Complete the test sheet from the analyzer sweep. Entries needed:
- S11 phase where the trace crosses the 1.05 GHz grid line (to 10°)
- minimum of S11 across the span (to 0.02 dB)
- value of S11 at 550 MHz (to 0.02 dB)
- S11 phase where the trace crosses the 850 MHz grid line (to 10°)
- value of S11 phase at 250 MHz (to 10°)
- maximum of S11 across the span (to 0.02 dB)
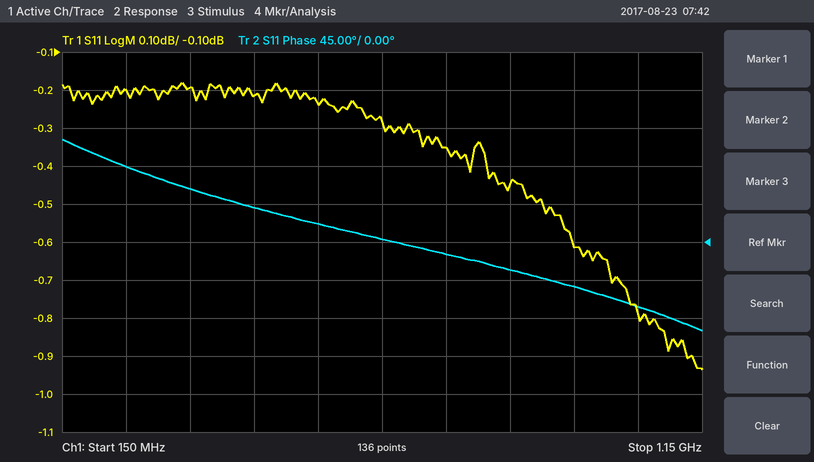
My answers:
-80°
-0.94 dB
-0.24 dB
-30°
90°
-0.18 dB
